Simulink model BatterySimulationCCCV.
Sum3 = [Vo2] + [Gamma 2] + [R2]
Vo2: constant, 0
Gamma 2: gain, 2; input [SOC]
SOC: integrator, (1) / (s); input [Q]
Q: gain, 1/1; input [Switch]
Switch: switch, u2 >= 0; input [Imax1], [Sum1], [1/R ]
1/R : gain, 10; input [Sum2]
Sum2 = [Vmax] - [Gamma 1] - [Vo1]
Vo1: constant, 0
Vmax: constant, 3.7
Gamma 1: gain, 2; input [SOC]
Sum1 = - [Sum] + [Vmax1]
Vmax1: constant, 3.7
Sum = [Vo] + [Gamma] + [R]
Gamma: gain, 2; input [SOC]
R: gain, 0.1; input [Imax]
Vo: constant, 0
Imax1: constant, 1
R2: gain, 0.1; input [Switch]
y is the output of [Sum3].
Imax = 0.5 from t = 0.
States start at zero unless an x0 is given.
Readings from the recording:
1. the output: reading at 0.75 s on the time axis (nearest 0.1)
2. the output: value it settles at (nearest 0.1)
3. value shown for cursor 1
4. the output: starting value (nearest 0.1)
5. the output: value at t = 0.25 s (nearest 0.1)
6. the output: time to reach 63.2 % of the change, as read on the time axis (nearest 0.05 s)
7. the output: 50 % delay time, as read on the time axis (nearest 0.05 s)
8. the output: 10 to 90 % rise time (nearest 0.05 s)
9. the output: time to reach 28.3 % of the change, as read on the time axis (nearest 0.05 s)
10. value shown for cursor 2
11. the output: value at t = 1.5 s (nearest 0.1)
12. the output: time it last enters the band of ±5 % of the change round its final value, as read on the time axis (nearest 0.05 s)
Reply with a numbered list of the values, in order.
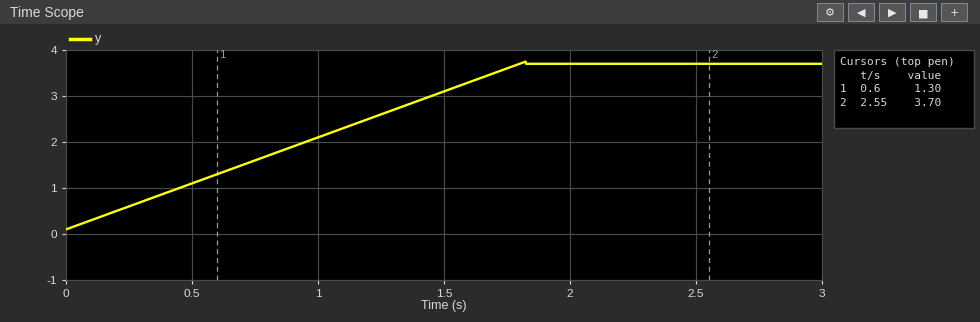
1. 1.6
2. 3.7
3. 1.30
4. 0.1
5. 0.6
6. 1.15 s
7. 0.90 s
8. 1.45 s
9. 0.50 s
10. 3.70
11. 3.1
12. 1.70 s
